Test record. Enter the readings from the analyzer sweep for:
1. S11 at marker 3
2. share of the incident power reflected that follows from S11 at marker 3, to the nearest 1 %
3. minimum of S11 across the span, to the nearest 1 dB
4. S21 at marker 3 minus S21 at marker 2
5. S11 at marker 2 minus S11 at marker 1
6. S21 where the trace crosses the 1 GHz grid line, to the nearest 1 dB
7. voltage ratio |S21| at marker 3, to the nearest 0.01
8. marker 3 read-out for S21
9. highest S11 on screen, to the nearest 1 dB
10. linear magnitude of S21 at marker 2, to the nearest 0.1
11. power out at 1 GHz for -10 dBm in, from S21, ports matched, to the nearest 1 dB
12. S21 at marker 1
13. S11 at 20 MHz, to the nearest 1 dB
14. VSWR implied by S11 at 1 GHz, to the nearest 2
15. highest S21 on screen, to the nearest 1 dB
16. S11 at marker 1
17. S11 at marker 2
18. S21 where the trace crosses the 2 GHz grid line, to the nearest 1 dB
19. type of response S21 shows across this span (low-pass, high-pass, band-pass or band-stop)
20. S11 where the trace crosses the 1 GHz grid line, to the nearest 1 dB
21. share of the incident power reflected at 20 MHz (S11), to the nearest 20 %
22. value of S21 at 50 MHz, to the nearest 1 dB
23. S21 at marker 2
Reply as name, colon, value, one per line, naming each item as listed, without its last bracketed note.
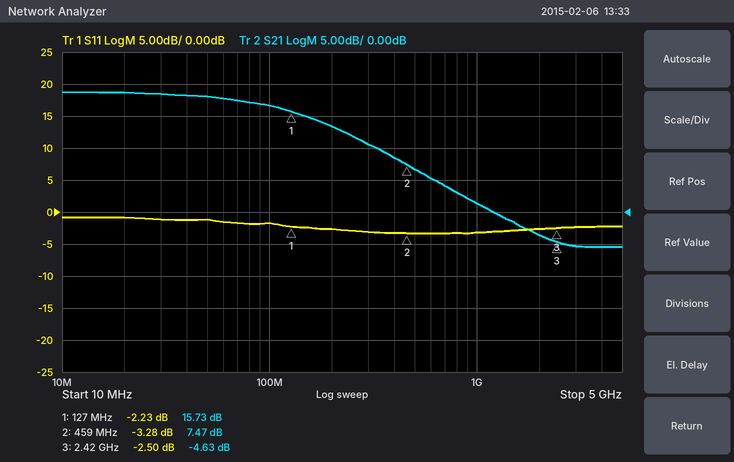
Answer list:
S11 at marker 3: -2.50 dB
share of the incident power reflected that follows from S11 at marker 3, to the nearest 1 %: 56 %
minimum of S11 across the span, to the nearest 1 dB: -3 dB
S21 at marker 3 minus S21 at marker 2: -12.10 dB
S11 at marker 2 minus S11 at marker 1: -1.05 dB
S21 where the trace crosses the 1 GHz grid line, to the nearest 1 dB: 1 dB
voltage ratio |S21| at marker 3, to the nearest 0.01: 0.59
marker 3 read-out for S21: -4.63 dB
highest S11 on screen, to the nearest 1 dB: -1 dB
linear magnitude of S21 at marker 2, to the nearest 0.1: 2.4
power out at 1 GHz for -10 dBm in, from S21, ports matched, to the nearest 1 dB: -9 dBm
S21 at marker 1: 15.73 dB
S11 at 20 MHz, to the nearest 1 dB: -1 dB
VSWR implied by S11 at 1 GHz, to the nearest 2: 6
highest S21 on screen, to the nearest 1 dB: 19 dB
S11 at marker 1: -2.23 dB
S11 at marker 2: -3.28 dB
S21 where the trace crosses the 2 GHz grid line, to the nearest 1 dB: -4 dB
type of response S21 shows across this span: low-pass
S11 where the trace crosses the 1 GHz grid line, to the nearest 1 dB: -3 dB
share of the incident power reflected at 20 MHz (S11), to the nearest 20 %: 80 %
value of S21 at 50 MHz, to the nearest 1 dB: 18 dB
S21 at marker 2: 7.47 dB
